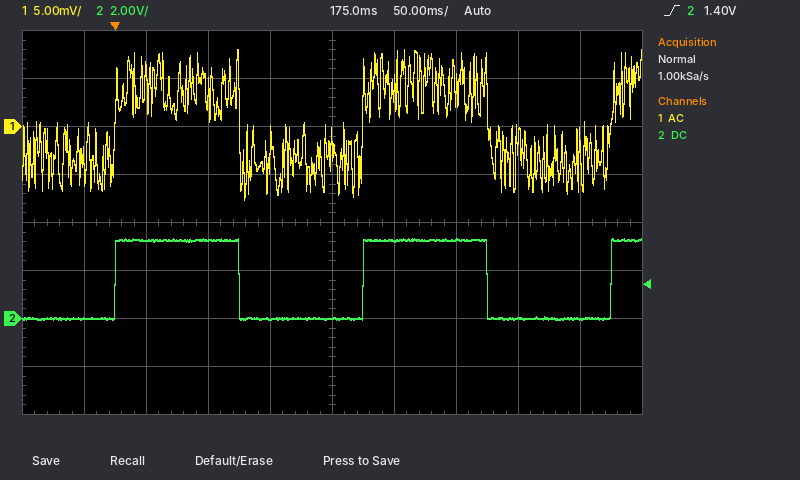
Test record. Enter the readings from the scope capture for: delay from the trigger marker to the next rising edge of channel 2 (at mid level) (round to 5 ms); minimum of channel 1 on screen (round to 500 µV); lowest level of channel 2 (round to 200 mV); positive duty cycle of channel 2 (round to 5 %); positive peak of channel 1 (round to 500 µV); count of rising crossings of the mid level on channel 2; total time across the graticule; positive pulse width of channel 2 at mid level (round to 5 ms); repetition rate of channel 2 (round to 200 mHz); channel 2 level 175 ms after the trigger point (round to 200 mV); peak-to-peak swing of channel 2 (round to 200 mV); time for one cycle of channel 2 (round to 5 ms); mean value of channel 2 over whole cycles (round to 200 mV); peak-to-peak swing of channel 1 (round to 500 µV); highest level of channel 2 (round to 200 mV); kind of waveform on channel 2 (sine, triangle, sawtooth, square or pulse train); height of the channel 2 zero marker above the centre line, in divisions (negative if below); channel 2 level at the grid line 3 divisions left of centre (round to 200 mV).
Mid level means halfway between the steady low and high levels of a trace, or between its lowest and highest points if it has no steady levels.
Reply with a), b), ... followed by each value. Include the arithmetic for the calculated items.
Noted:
a) 200 ms
b) -7.5 mV
c) 0.0 V
d) 100 ms / 200 ms ≈ 50 %
e) 8.0 mV
f) 3
g) 500 ms
h) 100 ms
i) 1 / 200 ms ≈ 5.0 Hz
j) 0.0 V
k) 3.4 V − (0.0 V) = 3.4 V
l) 200 ms
m) 0.0 V + 0.5 × (3.4 V − (0.0 V)) ≈ 1.70 V, so 1.6 V to the nearest 200 mV
n) 8.0 mV − (-7.5 mV) = 15.5 mV
o) 3.4 V
p) square
q) -2.0 div
r) 3.2 V
